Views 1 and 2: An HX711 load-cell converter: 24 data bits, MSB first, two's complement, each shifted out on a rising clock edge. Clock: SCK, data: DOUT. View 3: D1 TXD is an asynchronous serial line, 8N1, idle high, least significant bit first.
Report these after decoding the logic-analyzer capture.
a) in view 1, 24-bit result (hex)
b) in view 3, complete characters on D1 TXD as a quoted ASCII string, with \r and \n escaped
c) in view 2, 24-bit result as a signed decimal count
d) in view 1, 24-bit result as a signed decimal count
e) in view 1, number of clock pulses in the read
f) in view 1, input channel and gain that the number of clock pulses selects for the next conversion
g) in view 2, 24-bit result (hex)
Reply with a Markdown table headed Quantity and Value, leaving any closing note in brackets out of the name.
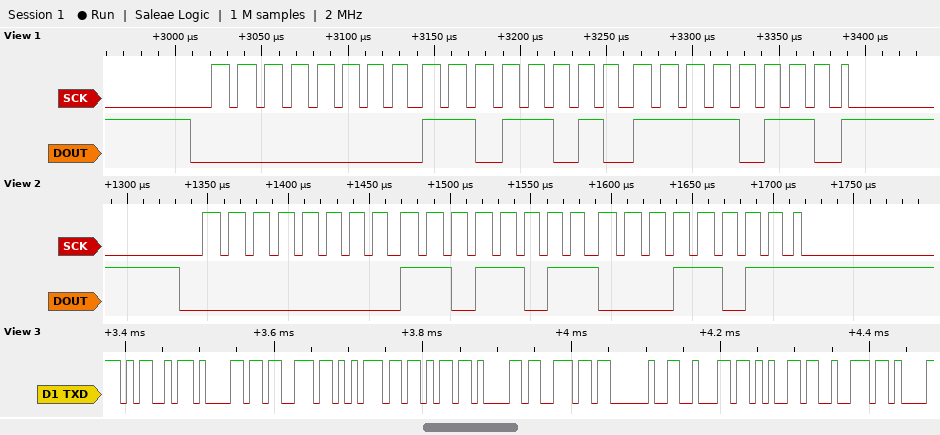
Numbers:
| Quantity | Value |
|---|---|
| in view 1, 24-bit result | 0x00DAF6 |
| in view 3, complete characters on D1 TXD as a quoted ASCII string, with \r and \n escaped | "Masukan ber" |
| in view 2, 24-bit result as a signed decimal count | 56091 |
| in view 1, 24-bit result as a signed decimal count | 56054 |
| in view 1, number of clock pulses in the read | 25 |
| in view 1, input channel and gain that the number of clock pulses selects for the next conversion | channel A, gain 128 |
| in view 2, 24-bit result | 0x00DB1B |
